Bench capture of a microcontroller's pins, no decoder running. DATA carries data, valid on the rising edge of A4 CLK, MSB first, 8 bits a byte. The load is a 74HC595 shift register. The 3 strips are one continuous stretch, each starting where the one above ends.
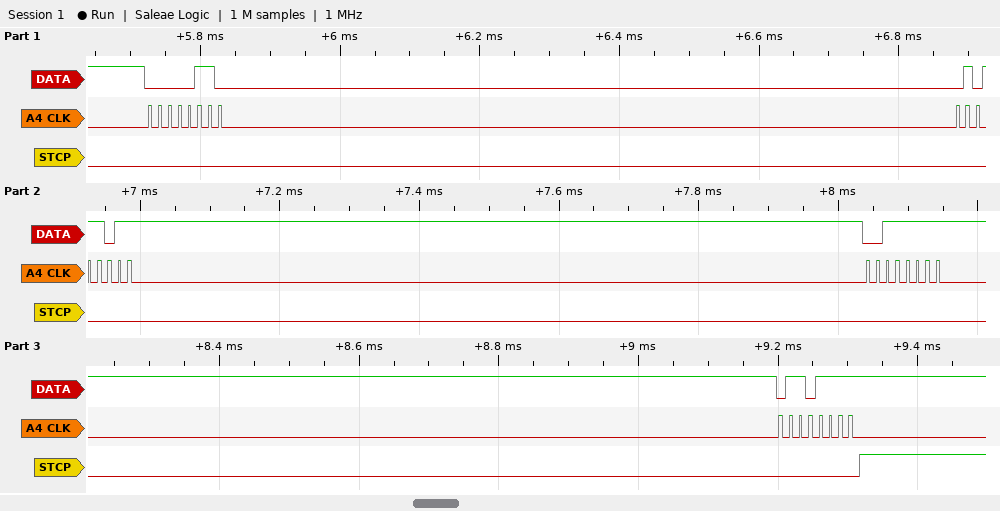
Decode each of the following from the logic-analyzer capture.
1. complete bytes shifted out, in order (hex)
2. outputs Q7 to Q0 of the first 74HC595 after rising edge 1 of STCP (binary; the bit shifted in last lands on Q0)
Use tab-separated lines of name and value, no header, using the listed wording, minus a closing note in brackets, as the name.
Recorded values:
complete bytes shifted out, in order	0x06 0x5B 0x3F 0x6F
outputs Q7 to Q0 of the first 74HC595 after rising edge 1 of STCP	01101111
